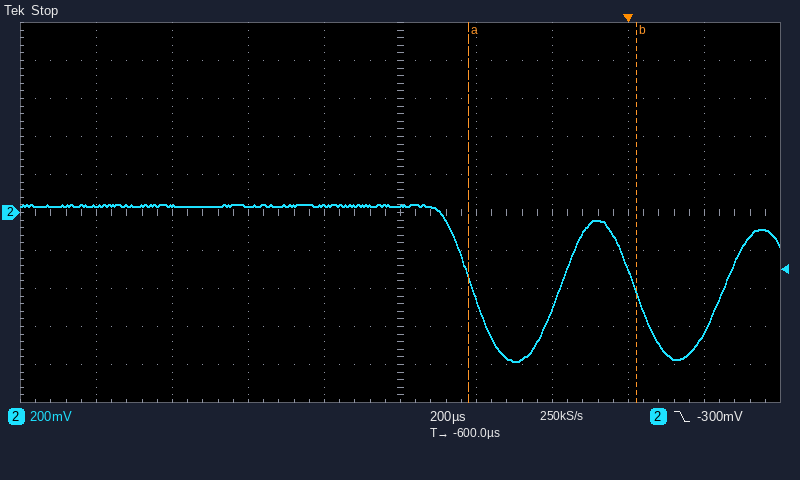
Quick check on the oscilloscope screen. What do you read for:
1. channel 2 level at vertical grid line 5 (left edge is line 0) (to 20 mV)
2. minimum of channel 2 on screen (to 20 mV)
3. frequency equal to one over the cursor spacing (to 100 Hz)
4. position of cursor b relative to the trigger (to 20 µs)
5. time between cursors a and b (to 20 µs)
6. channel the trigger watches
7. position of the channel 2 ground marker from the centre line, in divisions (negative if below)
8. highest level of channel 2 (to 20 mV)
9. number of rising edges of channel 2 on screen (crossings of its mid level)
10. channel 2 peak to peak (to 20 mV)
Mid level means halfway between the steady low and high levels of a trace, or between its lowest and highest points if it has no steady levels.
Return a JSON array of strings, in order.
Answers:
["40 mV", "-780 mV", "2.3 kHz", "+20 µs", "440 µs", "channel 2", "0.0 div", "40 mV", "2", "820 mV"]
